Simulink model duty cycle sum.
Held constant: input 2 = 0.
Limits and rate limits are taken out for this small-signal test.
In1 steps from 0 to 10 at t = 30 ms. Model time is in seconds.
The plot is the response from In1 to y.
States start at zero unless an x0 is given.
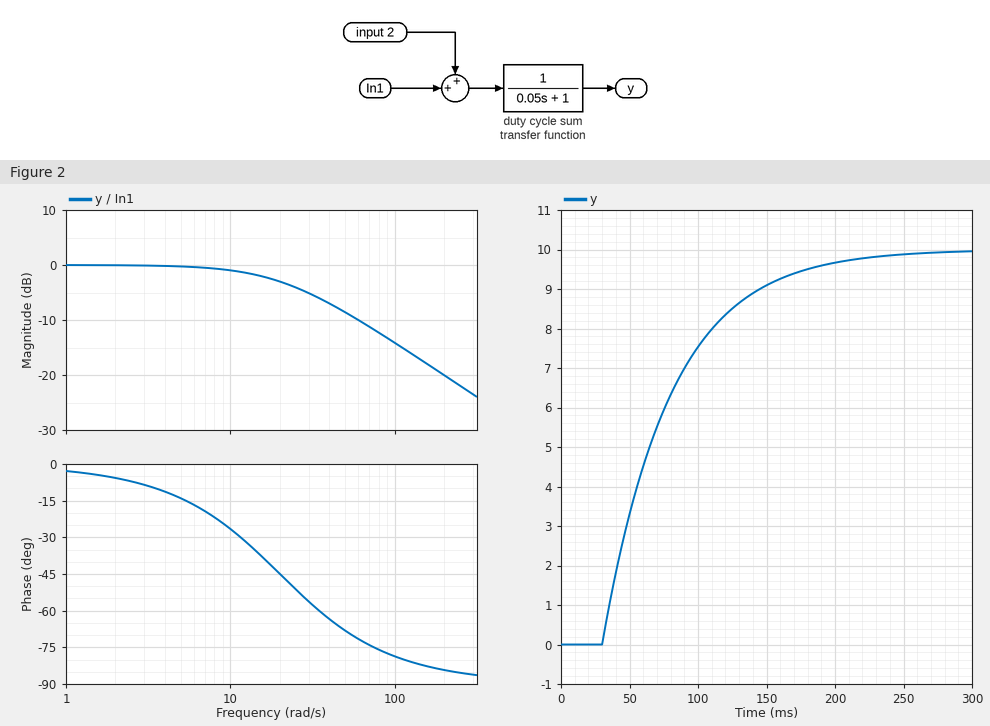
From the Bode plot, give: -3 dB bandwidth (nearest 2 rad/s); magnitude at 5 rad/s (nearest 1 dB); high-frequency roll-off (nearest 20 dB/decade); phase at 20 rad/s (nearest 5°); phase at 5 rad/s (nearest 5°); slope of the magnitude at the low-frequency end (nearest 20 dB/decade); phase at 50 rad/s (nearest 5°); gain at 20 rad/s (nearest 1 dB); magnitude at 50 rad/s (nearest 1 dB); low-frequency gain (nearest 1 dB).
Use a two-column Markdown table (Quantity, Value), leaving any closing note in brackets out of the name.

| Quantity | Value |
|---|---|
| -3 dB bandwidth | 20 rad/s |
| magnitude at 5 rad/s | 0 dB |
| high-frequency roll-off | -20 dB/decade |
| phase at 20 rad/s | -45° |
| phase at 5 rad/s | -15° |
| slope of the magnitude at the low-frequency end | 0 dB/decade |
| phase at 50 rad/s | -70° |
| gain at 20 rad/s | -3 dB |
| magnitude at 50 rad/s | -9 dB |
| low-frequency gain | 0 dB |
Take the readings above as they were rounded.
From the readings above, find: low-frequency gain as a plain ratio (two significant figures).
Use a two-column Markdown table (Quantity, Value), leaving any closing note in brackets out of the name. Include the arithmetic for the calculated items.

| Quantity | Value |
|---|---|
| low-frequency gain as a plain ratio | 10^(0 / 20) = 1.0 |
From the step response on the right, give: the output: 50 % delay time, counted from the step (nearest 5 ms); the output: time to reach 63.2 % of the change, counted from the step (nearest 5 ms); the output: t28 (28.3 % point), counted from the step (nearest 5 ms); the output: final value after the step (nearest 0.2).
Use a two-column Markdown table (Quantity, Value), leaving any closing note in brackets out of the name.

| Quantity | Value |
|---|---|
| the output: 50 % delay time, counted from the step | 35 ms |
| the output: time to reach 63.2 % of the change, counted from the step | 50 ms |
| the output: t28 (28.3 % point), counted from the step | 15 ms |
| the output: final value after the step | 10.0 |
